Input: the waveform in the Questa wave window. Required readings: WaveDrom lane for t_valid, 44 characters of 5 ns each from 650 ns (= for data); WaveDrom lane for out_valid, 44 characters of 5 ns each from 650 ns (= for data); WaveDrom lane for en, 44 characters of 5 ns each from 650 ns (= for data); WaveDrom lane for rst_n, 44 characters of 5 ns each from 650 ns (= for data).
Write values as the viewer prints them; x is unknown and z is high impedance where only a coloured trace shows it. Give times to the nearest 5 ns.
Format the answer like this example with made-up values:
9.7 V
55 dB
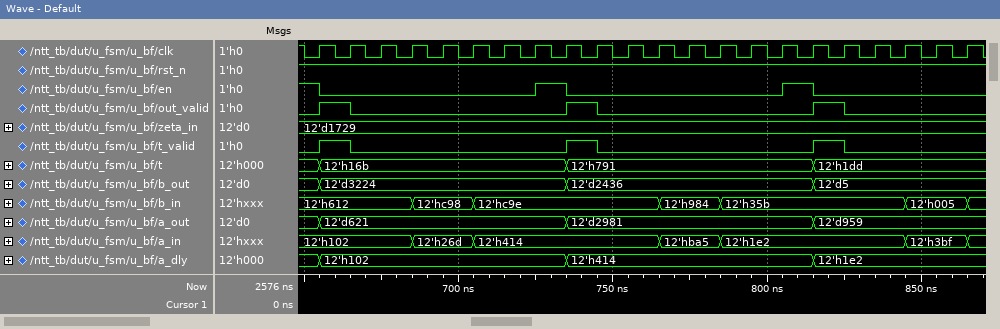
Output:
{name: 't_valid', wave: '01.0.............1.0.............1.0........'}
{name: 'out_valid', wave: '01.0.............1.0.............1.0........'}
{name: 'en', wave: '10.............1.0.............1.0..........'}
{name: 'rst_n', wave: '1...........................................'}
